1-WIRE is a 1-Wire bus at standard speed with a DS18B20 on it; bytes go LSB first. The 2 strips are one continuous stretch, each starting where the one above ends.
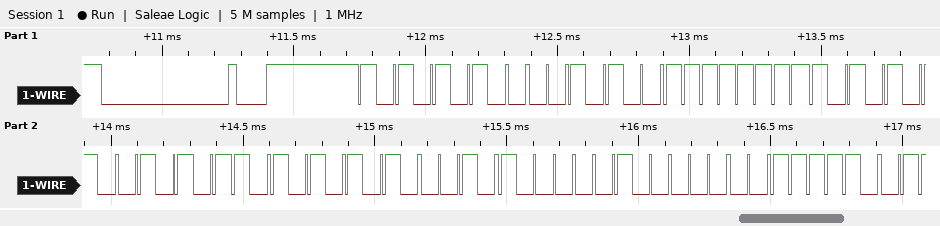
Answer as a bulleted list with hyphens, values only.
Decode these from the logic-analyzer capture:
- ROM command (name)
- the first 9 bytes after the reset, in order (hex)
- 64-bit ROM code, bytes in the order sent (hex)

- Match ROM
- 55 28 FF 55 6A 55 14 04 7C
- 28 FF 55 6A 55 14 04 7C
